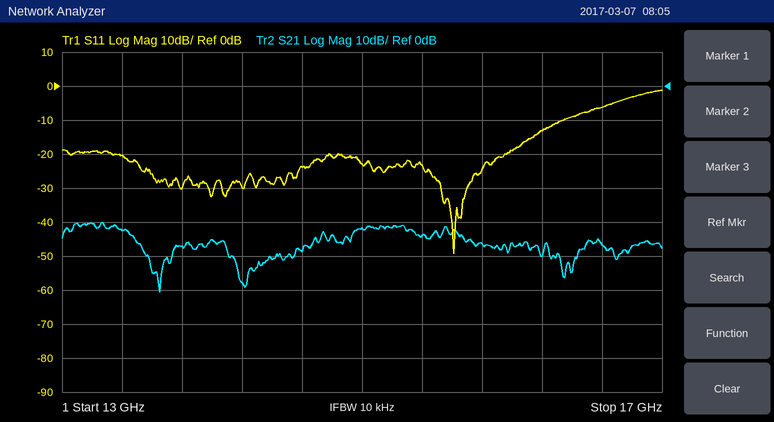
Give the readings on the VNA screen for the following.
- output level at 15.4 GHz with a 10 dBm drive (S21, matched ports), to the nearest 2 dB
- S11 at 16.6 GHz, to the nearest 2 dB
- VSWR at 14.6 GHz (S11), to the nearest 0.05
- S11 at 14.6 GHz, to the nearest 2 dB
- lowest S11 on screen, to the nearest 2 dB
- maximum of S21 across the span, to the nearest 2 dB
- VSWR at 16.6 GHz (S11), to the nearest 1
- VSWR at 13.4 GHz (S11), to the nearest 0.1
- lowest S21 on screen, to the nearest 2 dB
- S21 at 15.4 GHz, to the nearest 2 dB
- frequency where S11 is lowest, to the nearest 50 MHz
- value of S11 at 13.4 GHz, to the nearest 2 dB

-34 dBm
-6 dB
1.15
-24 dB
-50 dB
-40 dB
3
1.2
-60 dB
-44 dB
15.60 GHz
-20 dB
